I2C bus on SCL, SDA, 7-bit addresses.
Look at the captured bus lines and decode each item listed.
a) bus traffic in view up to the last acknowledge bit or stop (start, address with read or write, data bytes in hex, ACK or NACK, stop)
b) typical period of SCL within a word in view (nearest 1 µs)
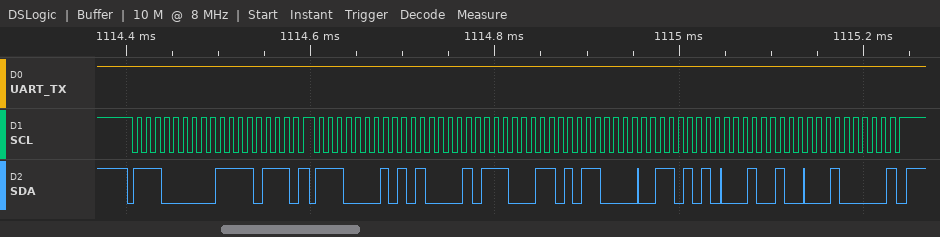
start, address 70 write ACK, F7 ACK, repeated start, address 70 read ACK, A1 ACK, E3 ACK, B0 ACK, 6A ACK, 24 ACK, 20 NACK, stop
10 µs
